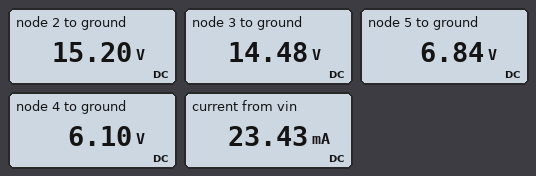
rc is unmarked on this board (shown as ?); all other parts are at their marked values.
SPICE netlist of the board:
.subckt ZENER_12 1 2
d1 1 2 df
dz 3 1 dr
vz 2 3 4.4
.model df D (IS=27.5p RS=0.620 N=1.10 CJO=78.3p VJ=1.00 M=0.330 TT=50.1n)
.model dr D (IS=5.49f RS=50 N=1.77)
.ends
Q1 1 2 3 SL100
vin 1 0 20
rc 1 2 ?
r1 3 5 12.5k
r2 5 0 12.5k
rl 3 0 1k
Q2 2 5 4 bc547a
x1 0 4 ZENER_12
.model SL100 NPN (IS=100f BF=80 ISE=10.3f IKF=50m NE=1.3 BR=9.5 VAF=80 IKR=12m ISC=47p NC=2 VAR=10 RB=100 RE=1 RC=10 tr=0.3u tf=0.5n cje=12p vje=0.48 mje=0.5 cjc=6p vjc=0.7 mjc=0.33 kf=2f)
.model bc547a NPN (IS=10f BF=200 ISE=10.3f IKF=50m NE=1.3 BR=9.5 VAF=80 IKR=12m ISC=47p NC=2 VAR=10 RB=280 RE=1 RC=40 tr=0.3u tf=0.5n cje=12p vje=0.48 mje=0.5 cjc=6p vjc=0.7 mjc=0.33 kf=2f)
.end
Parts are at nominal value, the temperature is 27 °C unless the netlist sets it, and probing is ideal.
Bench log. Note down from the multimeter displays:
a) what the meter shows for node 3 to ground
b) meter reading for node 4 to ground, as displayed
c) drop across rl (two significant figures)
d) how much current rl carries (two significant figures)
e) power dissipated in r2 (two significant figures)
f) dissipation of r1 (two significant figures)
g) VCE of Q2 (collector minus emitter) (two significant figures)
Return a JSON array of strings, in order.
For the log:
["14.48 V", "6.10 V", "14 V", "14 mA", "3.7 mW", "4.7 mW", "9.1 V"]
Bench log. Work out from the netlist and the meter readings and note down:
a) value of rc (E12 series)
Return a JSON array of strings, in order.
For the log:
["560 Ω"]
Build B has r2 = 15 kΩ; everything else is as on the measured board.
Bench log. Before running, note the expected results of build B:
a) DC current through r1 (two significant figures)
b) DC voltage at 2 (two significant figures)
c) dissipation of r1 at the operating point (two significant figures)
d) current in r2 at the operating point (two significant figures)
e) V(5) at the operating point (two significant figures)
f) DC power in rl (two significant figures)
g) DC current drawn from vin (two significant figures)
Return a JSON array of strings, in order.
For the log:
["540 µA", "14 V", "3.6 mW", "460 µA", "6.9 V", "190 mW", "24 mA"]
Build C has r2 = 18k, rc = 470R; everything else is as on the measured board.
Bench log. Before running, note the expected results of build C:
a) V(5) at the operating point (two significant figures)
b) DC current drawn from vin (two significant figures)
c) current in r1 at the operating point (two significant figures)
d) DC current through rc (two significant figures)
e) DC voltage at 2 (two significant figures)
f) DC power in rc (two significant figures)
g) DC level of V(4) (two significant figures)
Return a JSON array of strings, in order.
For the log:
["7.1 V", "26 mA", "500 µA", "13 mA", "14 V", "76 mW", "6.3 V"]
